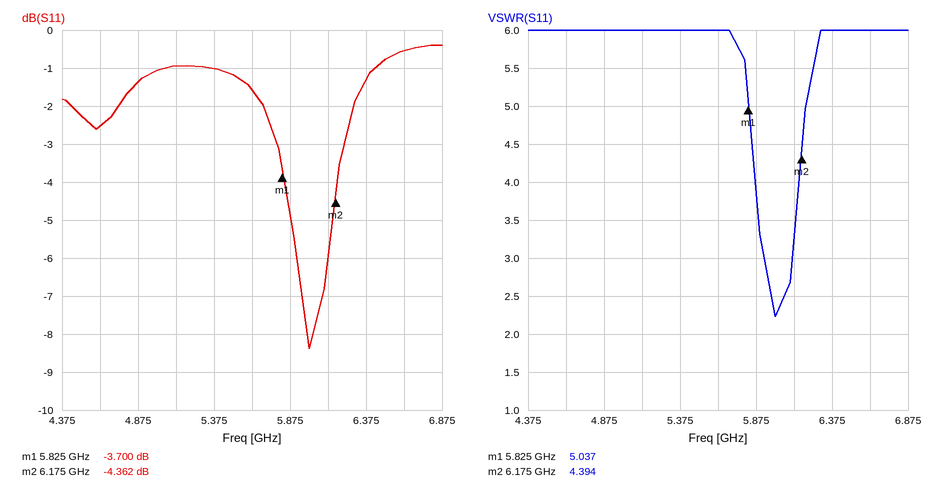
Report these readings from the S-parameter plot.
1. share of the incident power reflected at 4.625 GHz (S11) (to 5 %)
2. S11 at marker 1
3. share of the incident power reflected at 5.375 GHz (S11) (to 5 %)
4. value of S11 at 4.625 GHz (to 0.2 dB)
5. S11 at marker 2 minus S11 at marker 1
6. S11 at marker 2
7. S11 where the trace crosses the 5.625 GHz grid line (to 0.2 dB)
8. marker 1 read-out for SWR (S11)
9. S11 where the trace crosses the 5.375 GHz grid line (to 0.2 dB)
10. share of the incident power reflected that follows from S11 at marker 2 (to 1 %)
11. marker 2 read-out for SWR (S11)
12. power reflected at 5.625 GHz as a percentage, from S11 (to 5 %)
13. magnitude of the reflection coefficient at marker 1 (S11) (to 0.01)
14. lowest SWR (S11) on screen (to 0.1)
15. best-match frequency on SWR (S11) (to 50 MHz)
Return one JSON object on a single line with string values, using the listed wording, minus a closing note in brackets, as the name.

{"share of the incident power reflected at 4.625 GHz (S11)": "55 %", "S11 at marker 1": "-3.700 dB", "share of the incident power reflected at 5.375 GHz (S11)": "80 %", "value of S11 at 4.625 GHz": "-2.6 dB", "S11 at marker 2 minus S11 at marker 1": "-0.662 dB", "S11 at marker 2": "-4.362 dB", "S11 where the trace crosses the 5.625 GHz grid line": "-1.6 dB", "marker 1 read-out for SWR": "5.037", "S11 where the trace crosses the 5.375 GHz grid line": "-1.0 dB", "share of the incident power reflected that follows from S11 at marker 2": "37 %", "marker 2 read-out for SWR": "4.394", "power reflected at 5.625 GHz as a percentage, from S11": "70 %", "magnitude of the reflection coefficient at marker 1 (S11)": "0.65", "lowest SWR (S11) on screen": "2.2", "best-match frequency on SWR (S11)": "6.00 GHz"}
